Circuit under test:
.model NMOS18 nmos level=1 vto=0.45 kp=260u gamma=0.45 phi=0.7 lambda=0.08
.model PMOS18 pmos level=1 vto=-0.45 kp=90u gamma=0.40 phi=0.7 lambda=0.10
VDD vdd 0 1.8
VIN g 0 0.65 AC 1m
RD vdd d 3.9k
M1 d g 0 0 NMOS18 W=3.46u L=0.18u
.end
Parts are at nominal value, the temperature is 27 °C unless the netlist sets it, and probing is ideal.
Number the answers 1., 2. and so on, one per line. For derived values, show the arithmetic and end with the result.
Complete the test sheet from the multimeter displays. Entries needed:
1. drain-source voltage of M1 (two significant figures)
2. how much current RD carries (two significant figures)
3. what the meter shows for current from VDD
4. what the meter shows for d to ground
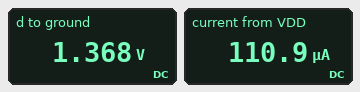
1. 1.368 V = 1.4 V
2. (1.8 V - 1.368 V) / 3.9 kΩ = 110 µA
3. 110.9 µA
4. 1.368 V
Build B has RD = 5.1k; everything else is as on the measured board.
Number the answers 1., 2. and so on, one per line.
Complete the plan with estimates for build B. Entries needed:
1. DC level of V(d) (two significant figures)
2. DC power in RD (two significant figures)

1. 1.2 V
2. 62 µW
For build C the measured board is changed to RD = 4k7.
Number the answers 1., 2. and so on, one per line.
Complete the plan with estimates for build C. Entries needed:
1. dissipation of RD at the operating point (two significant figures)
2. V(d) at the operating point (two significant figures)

1. 57 µW
2. 1.3 V
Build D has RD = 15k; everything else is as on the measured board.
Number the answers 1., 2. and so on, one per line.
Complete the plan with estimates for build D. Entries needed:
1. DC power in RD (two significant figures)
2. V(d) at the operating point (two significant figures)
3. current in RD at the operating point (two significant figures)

1. 160 µW
2. 270 mV
3. 100 µA
